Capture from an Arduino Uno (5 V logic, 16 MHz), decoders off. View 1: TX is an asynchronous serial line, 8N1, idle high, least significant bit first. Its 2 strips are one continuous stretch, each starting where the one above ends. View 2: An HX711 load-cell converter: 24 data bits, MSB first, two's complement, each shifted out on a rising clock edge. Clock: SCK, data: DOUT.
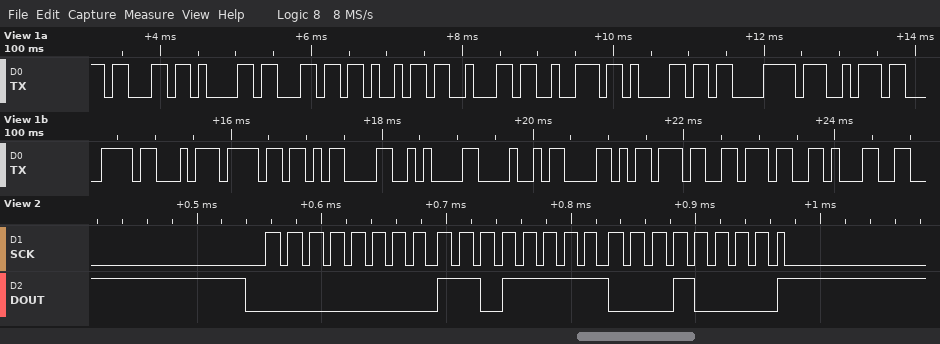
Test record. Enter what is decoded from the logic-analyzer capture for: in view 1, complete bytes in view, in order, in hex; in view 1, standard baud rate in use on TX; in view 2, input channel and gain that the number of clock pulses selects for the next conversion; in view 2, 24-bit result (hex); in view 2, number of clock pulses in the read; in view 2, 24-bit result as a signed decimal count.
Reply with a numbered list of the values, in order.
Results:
1. 63 61 6C 69 62 72 61 C3 A7 C3 A3 6F 0D 0A 48 58 37 37 31
2. 9600 baud
3. channel A, gain 128
4. 0x00DF10
5. 25
6. 57104
